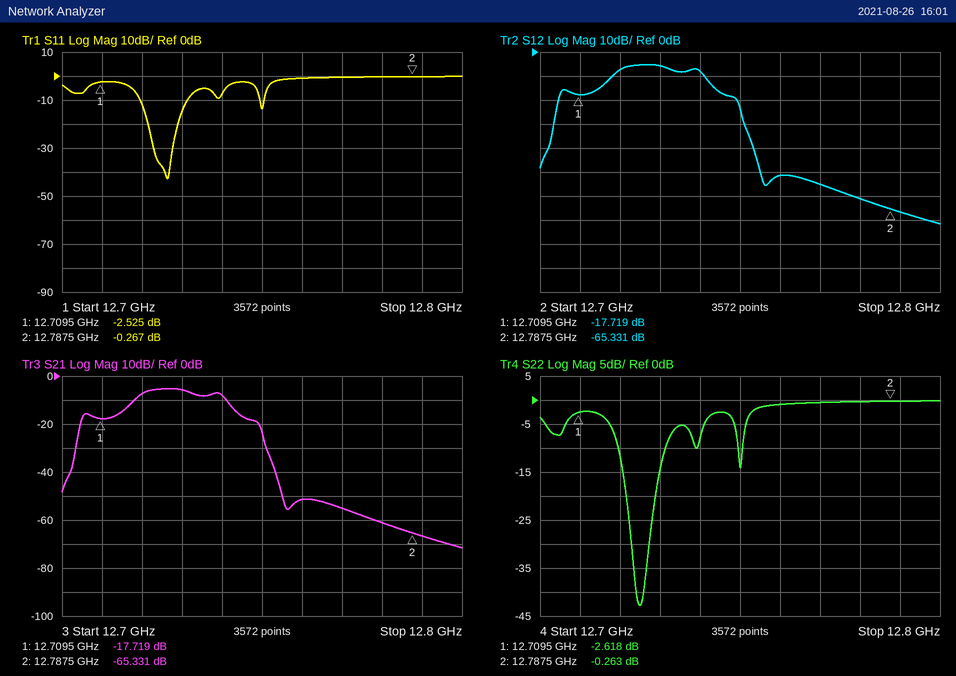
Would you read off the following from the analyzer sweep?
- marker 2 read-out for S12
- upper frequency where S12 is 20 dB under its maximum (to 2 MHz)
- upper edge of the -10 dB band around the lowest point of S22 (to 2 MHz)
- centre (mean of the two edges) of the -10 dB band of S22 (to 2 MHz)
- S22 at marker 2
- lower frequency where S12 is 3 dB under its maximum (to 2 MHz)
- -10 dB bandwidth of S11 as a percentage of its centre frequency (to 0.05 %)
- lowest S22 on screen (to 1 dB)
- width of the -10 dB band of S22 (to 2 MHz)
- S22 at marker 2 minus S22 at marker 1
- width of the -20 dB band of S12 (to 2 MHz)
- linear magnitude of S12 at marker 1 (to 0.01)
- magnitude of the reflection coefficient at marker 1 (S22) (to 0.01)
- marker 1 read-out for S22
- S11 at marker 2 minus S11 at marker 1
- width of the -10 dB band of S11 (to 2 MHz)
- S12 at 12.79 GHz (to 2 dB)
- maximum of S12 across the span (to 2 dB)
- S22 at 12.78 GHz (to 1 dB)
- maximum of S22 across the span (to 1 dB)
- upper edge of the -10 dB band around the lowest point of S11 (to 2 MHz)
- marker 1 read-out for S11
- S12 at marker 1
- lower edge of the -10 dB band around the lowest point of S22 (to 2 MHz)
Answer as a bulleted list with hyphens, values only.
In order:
- -65.331 dB
- 12.750 GHz
- 12.732 GHz
- 12.726 GHz
- -0.263 dB
- 12.720 GHz
- 0.10 %
- -43 dB
- 12 MHz
- 2.355 dB
- 46 MHz
- 0.13
- 0.74
- -2.618 dB
- 2.258 dB
- 12 MHz
- -66 dB
- -6 dB
- 0 dB
- 0 dB
- 12.732 GHz
- -2.525 dB
- -17.719 dB
- 12.720 GHz
